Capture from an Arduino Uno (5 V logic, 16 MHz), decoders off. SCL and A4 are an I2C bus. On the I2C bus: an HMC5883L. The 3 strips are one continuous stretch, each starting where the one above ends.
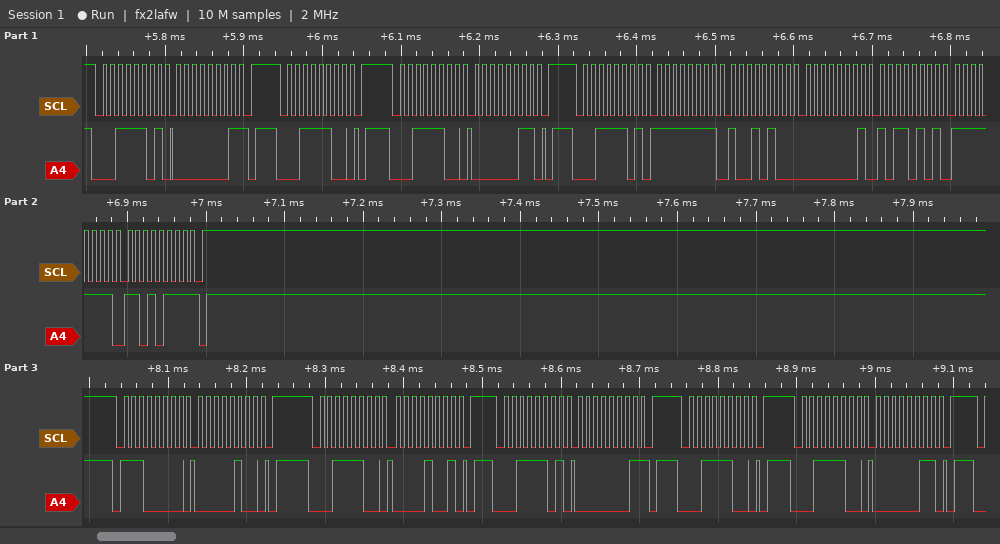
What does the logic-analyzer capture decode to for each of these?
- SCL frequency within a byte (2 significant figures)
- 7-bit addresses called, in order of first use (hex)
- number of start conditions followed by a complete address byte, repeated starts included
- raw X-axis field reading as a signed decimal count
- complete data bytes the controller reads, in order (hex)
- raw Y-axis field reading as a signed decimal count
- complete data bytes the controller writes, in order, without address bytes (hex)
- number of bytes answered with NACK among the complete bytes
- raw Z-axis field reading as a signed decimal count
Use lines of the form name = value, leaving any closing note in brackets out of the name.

SCL frequency within a byte = 100 kHz
7-bit addresses called, in order of first use = 0x1E 0x70
number of start conditions followed by a complete address byte, repeated starts included = 9
raw X-axis field reading as a signed decimal count = -108
complete data bytes the controller reads, in order = 01 FF 94 01 B5 FF D7 01
raw Y-axis field reading as a signed decimal count = -41
complete data bytes the controller writes, in order, without address bytes = 03 04 09 03
number of bytes answered with NACK among the complete bytes = 3
raw Z-axis field reading as a signed decimal count = 437
